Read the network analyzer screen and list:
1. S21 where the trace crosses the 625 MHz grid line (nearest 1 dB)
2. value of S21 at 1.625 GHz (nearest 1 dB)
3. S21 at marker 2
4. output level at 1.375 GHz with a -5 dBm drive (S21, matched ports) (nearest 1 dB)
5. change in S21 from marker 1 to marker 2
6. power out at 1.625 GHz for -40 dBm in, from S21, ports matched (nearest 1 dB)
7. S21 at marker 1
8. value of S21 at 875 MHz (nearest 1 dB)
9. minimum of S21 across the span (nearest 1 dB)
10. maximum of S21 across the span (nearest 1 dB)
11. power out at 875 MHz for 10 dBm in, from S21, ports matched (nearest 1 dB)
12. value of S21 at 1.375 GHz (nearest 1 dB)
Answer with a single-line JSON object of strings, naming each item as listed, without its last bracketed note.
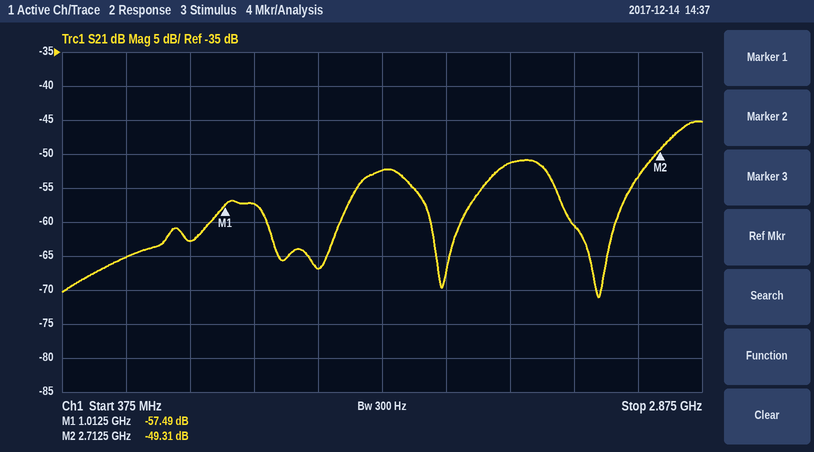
{"S21 where the trace crosses the 625 MHz grid line": "-65 dB", "value of S21 at 1.625 GHz": "-52 dB", "S21 at marker 2": "-49.31 dB", "output level at 1.375 GHz with a -5 dBm drive (S21, matched ports)": "-72 dBm", "change in S21 from marker 1 to marker 2": "8.18 dB", "power out at 1.625 GHz for -40 dBm in, from S21, ports matched": "-92 dBm", "S21 at marker 1": "-57.49 dB", "value of S21 at 875 MHz": "-63 dB", "minimum of S21 across the span": "-71 dB", "maximum of S21 across the span": "-45 dB", "power out at 875 MHz for 10 dBm in, from S21, ports matched": "-53 dBm", "value of S21 at 1.375 GHz": "-67 dB"}
